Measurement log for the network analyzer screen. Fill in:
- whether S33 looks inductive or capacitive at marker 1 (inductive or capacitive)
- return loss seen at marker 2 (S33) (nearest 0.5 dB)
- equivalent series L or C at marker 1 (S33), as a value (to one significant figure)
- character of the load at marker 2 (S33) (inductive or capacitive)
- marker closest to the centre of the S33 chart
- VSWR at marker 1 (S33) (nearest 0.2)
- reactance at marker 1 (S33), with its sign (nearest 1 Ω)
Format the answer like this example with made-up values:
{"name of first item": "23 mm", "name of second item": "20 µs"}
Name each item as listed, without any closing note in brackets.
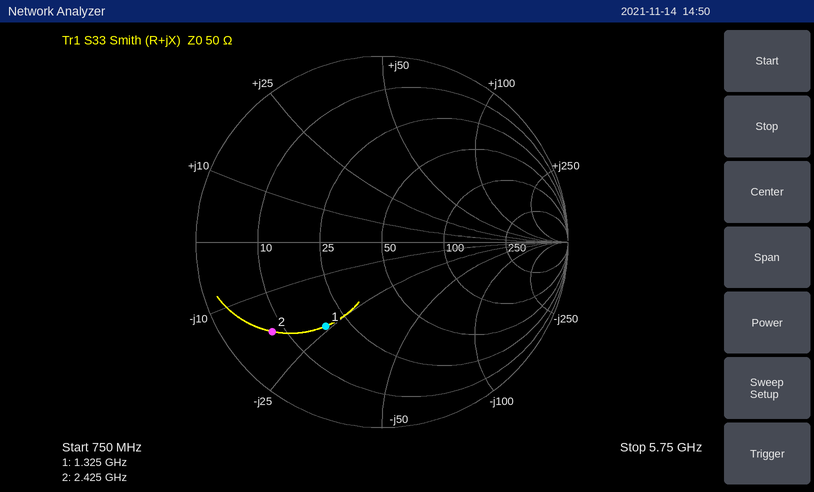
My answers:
{"whether S33 looks inductive or capacitive at marker 1": "capacitive", "return loss seen at marker 2 (S33)": "2.5 dB", "equivalent series L or C at marker 1 (S33), as a value": "5 pF", "character of the load at marker 2 (S33)": "capacitive", "marker closest to the centre of the S33 chart": "marker 1", "VSWR at marker 1 (S33)": "3.4", "reactance at marker 1 (S33), with its sign": "-24 Ω"}
